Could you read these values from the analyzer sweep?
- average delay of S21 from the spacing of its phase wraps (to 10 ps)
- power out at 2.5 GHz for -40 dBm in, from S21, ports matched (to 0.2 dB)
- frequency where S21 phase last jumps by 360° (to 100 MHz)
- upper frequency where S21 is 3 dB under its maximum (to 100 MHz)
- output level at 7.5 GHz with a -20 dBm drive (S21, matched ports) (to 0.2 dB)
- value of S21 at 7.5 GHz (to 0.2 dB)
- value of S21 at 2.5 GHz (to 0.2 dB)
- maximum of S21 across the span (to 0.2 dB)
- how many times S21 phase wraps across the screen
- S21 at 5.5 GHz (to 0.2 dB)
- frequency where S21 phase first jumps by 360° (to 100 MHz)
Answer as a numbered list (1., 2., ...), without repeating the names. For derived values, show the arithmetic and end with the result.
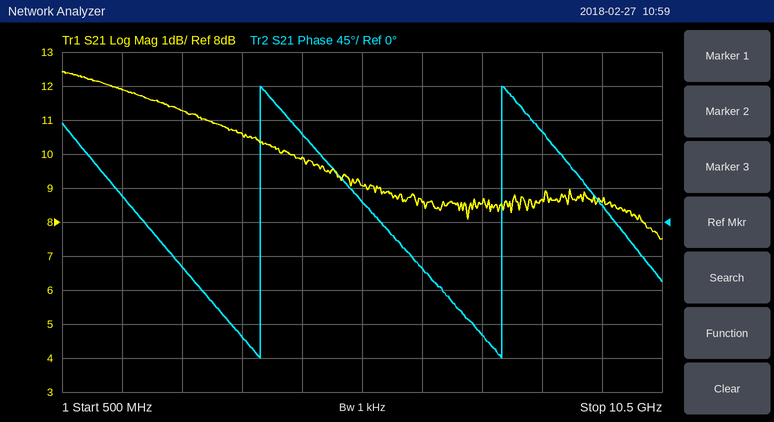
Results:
1. 1 cycle / (7.8 GHz − 3.8 GHz) ≈ 250 ps
2. -40 dBm + (11.2 dB) = -28.8 dBm
3. 7.8 GHz
4. 5.1 GHz
5. -20 dBm + (8.6 dB) = -11.4 dBm
6. 8.6 dB
7. 11.2 dB
8. 12.4 dB
9. 2
10. 9.0 dB
11. 3.8 GHz
